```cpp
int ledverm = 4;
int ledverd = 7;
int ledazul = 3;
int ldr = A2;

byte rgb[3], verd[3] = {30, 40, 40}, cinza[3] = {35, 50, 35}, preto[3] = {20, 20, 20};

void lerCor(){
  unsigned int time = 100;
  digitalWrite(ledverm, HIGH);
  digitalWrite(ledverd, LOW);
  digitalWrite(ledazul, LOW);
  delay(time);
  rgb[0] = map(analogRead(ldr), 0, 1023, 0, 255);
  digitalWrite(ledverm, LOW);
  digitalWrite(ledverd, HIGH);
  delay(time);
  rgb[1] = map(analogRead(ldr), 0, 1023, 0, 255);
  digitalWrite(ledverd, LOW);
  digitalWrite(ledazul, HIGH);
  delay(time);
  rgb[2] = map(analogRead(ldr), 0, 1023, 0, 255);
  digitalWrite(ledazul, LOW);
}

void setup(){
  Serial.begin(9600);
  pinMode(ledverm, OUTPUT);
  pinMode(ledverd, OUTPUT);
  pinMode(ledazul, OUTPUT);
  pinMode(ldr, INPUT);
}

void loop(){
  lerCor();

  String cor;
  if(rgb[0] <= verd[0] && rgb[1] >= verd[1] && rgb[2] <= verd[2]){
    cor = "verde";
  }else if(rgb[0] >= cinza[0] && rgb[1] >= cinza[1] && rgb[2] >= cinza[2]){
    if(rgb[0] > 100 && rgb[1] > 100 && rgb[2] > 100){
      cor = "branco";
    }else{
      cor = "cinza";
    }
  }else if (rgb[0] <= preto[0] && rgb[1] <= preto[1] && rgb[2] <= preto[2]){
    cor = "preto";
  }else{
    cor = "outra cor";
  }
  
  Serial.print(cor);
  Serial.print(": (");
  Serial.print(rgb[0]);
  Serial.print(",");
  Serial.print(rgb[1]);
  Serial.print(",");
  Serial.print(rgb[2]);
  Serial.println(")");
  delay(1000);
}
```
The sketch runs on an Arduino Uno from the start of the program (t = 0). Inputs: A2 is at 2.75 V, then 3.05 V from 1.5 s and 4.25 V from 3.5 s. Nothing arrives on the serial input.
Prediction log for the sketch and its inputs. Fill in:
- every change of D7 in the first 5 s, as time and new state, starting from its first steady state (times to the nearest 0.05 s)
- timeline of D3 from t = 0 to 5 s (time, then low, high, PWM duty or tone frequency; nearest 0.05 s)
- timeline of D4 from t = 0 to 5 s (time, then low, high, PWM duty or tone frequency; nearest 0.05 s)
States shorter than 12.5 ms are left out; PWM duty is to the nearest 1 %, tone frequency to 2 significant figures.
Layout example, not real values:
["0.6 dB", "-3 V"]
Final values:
["0 s low; 0.1 s high; 0.2 s low; 1.4 s high; 1.5 s low; 2.7 s high; 2.8 s low; 4 s high; 4.1 s low", "0 s low; 0.2 s high; 0.3 s low; 1.5 s high; 1.6 s low; 2.8 s high; 2.9 s low; 4.1 s high; 4.2 s low", "0 s high; 0.1 s low; 1.3 s high; 1.4 s low; 2.6 s high; 2.7 s low; 3.9 s high; 4 s low"]
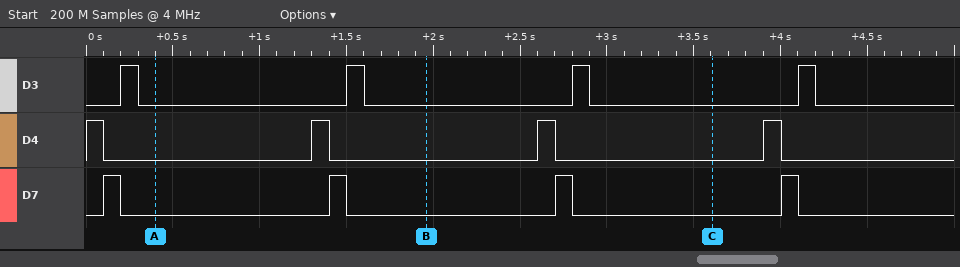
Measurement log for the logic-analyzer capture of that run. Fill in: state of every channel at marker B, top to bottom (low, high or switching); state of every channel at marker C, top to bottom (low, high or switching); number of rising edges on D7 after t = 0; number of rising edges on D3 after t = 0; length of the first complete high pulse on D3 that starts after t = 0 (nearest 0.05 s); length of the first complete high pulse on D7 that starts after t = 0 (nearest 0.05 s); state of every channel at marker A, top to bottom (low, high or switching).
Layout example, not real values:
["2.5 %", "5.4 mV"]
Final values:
["D3 low, D4 low, D7 low", "D3 low, D4 low, D7 low", "4", "4", "0.10 s", "0.10 s", "D3 low, D4 low, D7 low"]
